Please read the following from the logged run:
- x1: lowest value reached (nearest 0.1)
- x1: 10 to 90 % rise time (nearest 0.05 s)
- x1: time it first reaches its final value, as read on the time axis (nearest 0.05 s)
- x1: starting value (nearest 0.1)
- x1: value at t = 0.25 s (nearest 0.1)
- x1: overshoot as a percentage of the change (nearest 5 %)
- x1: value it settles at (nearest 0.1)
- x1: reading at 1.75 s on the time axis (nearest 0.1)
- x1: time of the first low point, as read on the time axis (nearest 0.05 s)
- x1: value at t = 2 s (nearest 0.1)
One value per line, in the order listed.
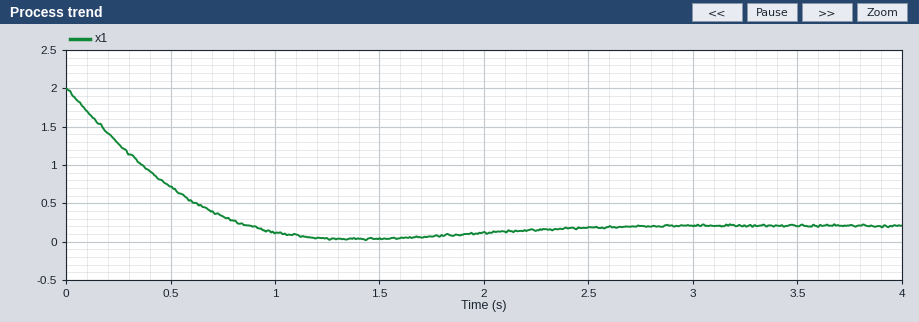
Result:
0.0
0.65 s
0.90 s
2.0
1.3
10 %
0.2
0.1
1.40 s
0.1
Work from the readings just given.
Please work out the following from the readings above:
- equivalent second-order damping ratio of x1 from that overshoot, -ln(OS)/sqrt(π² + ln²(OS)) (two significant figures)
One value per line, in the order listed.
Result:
0.59
